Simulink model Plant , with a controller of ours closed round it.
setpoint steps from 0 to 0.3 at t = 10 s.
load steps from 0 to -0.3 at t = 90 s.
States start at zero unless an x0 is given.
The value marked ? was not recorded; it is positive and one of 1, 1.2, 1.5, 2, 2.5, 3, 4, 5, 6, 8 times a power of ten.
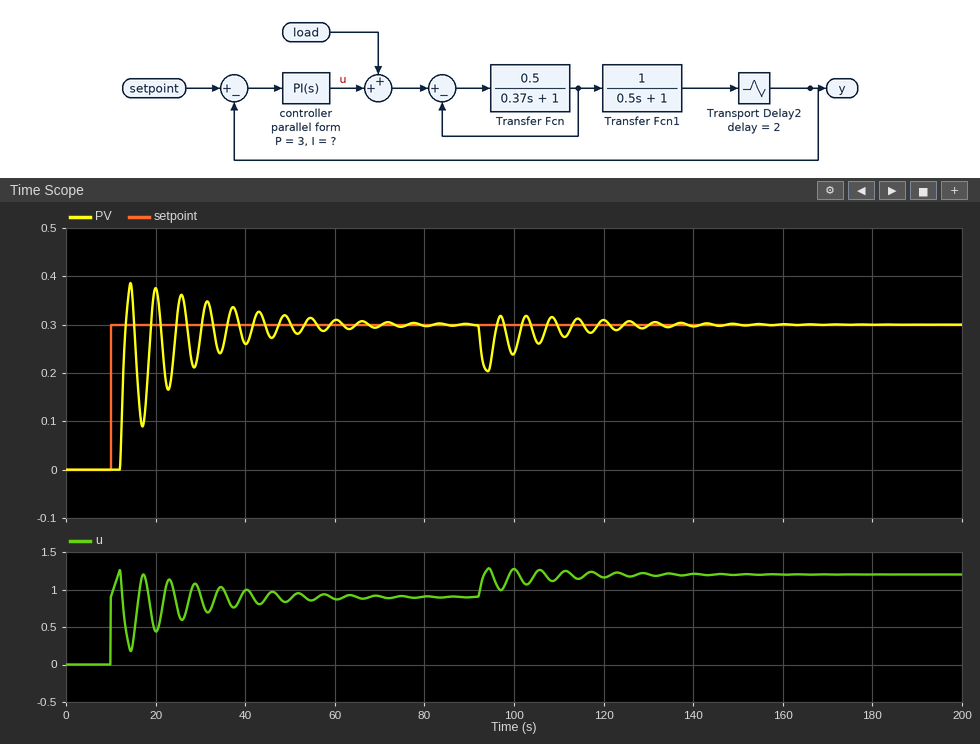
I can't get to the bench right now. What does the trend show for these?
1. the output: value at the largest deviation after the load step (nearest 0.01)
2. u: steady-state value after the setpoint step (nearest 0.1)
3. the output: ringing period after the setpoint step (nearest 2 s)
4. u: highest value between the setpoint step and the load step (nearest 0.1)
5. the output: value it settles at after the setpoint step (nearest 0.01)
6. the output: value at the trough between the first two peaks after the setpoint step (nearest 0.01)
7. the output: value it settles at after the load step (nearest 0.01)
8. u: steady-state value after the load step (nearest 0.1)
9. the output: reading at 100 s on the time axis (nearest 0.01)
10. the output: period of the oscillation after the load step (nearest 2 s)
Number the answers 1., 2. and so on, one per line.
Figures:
1. 0.20
2. 0.9
3. 6 s
4. 1.3
5. 0.30
6. 0.09
7. 0.30
8. 1.2
9. 0.24
10. 6 s
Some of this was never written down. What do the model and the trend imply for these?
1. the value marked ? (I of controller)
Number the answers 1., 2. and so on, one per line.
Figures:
1. 0.6
